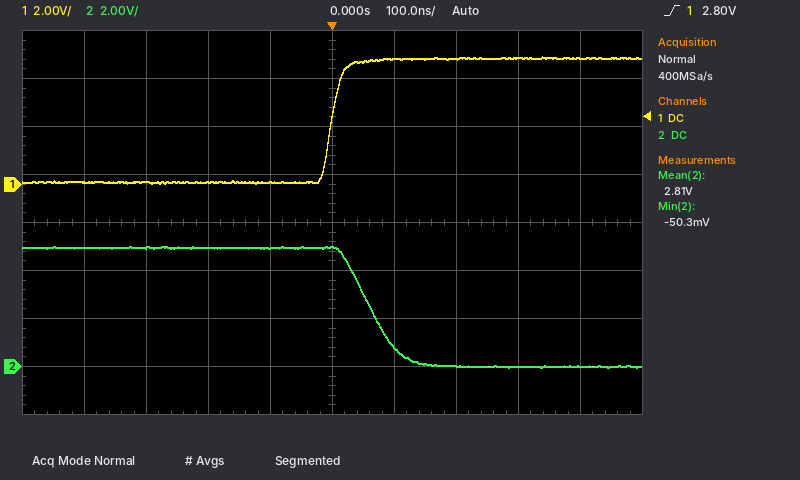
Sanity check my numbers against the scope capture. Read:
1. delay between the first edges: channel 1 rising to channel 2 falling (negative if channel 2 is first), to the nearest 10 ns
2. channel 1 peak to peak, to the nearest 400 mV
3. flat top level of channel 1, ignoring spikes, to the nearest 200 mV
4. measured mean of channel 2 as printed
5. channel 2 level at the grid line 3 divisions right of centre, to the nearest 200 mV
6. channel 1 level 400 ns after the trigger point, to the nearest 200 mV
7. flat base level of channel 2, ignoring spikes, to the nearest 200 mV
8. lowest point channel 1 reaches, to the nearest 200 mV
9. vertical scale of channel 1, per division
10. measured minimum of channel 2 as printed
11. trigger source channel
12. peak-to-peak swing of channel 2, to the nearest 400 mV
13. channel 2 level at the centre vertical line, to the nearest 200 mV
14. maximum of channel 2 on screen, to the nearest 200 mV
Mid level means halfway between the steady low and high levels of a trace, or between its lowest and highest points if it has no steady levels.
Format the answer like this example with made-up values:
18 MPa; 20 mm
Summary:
+60 ns; 5.2 V; 5.2 V; 2.81 V; 0.0 V; 5.2 V; 0.0 V; 0.0 V; 2 V; -50.3 mV; channel 1; 5.2 V; 5.0 V; 5.0 V
